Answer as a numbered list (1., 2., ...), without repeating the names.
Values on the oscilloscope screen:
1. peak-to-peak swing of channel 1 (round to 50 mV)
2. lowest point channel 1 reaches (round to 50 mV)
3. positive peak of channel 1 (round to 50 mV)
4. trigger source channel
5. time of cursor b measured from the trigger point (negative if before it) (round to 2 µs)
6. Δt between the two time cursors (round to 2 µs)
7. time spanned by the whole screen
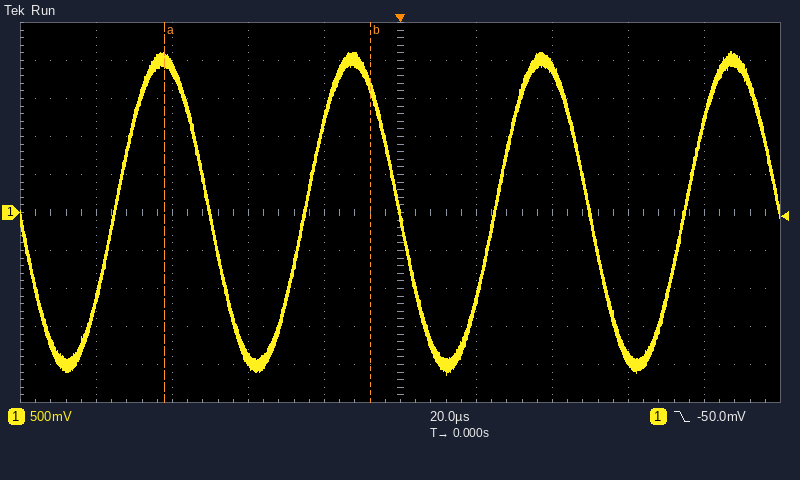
1. 4.25 V
2. -2.15 V
3. 2.10 V
4. channel 1
5. -8 µs
6. 54 µs
7. 200 µs
